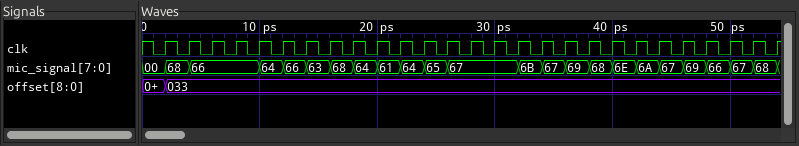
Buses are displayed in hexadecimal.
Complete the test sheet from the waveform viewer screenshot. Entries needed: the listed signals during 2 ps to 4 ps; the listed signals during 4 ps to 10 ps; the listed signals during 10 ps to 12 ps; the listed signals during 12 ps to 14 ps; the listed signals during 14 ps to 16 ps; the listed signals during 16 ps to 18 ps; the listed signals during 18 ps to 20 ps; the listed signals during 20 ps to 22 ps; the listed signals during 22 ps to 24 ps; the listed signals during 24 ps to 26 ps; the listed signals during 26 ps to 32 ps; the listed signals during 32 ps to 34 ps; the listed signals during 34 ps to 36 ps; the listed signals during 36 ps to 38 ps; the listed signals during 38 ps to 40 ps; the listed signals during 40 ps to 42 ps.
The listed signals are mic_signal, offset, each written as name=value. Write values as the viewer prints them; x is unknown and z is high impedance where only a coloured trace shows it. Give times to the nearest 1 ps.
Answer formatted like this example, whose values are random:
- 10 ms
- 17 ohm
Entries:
- mic_signal=68, offset=033
- mic_signal=66, offset=033
- mic_signal=64, offset=033
- mic_signal=66, offset=033
- mic_signal=63, offset=033
- mic_signal=68, offset=033
- mic_signal=64, offset=033
- mic_signal=61, offset=033
- mic_signal=64, offset=033
- mic_signal=65, offset=033
- mic_signal=67, offset=033
- mic_signal=6B, offset=033
- mic_signal=67, offset=033
- mic_signal=69, offset=033
- mic_signal=68, offset=033
- mic_signal=6E, offset=033
